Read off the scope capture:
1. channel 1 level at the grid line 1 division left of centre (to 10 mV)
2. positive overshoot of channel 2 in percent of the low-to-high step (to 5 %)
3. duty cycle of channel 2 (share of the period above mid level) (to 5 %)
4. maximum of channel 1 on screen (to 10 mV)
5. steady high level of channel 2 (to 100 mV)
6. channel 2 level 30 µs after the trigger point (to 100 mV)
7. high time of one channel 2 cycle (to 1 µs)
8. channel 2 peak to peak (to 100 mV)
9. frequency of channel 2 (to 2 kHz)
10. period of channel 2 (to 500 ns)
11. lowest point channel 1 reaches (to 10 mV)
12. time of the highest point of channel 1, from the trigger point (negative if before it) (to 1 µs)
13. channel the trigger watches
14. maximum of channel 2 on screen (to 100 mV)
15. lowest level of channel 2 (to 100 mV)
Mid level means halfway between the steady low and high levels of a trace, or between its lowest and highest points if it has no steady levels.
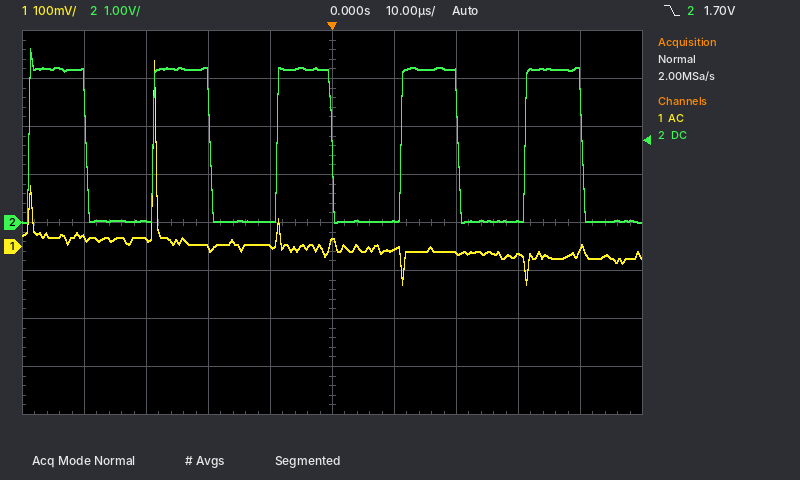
0 mV
15 %
45 %
390 mV
3.2 V
0.0 V
9 µs
3.6 V
50 kHz
20.0 µs
-80 mV
-29 µs
channel 2
3.6 V
0.0 V
